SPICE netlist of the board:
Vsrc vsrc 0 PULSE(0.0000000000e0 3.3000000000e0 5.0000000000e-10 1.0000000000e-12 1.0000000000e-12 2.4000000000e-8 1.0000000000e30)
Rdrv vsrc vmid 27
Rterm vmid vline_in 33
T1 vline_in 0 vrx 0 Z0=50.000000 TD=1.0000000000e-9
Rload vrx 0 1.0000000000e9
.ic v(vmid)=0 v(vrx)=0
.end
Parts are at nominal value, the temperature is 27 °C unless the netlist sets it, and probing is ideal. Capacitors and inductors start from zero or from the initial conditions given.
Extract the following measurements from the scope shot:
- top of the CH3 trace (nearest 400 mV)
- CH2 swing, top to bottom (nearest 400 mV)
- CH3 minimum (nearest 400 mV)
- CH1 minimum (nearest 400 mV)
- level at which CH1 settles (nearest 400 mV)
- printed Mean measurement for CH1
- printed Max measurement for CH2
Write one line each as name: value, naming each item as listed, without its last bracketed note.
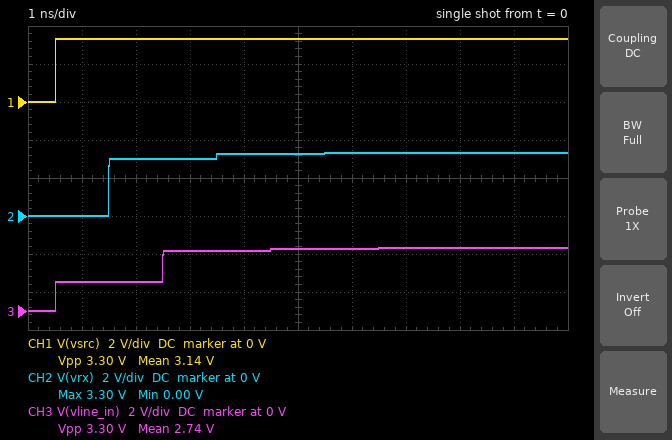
top of the CH3 trace: 3.2 V
CH2 swing, top to bottom: 3.2 V
CH3 minimum: 0 V
CH1 minimum: 0 V
level at which CH1 settles: 3.2 V
printed Mean measurement for CH1: 3.14 V
printed Max measurement for CH2: 3.30 V
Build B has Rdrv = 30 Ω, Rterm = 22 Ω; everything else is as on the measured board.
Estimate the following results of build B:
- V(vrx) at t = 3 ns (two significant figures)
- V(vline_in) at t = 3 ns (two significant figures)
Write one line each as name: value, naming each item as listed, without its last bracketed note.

V(vrx) at t = 3 ns: 3.2 V
V(vline_in) at t = 3 ns: 3.3 V
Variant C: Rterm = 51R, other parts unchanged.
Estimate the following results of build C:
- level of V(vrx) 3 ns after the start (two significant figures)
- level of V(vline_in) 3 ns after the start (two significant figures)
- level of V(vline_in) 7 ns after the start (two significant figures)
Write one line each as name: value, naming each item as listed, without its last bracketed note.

level of V(vrx) 3 ns after the start: 2.6 V
level of V(vline_in) 3 ns after the start: 2.9 V
level of V(vline_in) 7 ns after the start: 3.3 V
